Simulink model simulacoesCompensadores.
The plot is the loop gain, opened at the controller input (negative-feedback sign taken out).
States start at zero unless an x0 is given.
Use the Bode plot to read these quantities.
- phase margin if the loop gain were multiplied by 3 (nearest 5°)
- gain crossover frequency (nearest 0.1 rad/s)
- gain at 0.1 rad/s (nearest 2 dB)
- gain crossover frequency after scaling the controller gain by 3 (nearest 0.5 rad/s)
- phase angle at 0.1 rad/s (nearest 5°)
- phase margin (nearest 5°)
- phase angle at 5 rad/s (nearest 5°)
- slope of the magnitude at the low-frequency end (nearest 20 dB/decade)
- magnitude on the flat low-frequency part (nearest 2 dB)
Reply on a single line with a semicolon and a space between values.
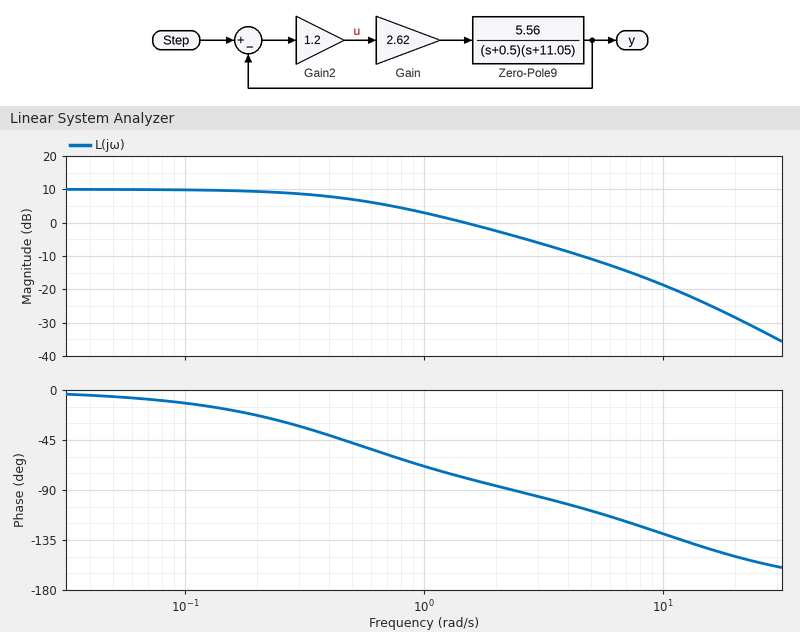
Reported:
75°; 1.5 rad/s; 10 dB; 4.5 rad/s; -10°; 100°; -110°; 0 dB/decade; 10 dB
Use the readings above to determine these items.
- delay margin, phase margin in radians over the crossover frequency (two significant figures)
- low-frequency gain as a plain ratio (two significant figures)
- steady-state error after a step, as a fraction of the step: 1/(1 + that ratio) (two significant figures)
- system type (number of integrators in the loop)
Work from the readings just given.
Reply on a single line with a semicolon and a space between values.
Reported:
1.2 s; 3.2; 0.24; 0
